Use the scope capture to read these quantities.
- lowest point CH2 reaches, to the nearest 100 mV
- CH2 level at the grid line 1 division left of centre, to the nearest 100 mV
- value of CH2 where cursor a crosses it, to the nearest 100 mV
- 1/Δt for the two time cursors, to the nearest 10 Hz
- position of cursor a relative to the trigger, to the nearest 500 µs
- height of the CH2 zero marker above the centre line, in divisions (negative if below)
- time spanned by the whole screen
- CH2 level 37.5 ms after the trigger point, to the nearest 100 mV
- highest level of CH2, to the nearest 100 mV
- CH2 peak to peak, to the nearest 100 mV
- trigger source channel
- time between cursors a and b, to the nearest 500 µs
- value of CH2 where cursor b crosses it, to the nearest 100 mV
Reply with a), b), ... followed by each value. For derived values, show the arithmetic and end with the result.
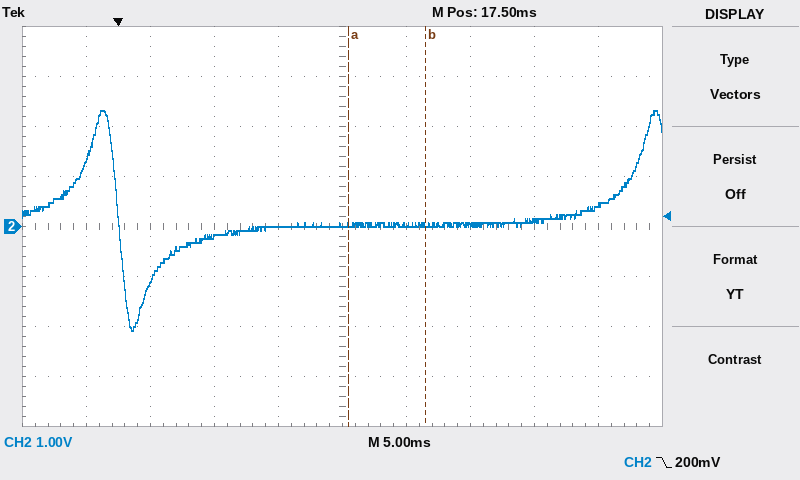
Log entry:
a) -2.1 V
b) 0.0 V
c) 0.0 V
d) 1 / 6.0 ms ≈ 170 Hz
e) +18.0 ms
f) 0.0 div
g) 50 ms
h) 400 mV
i) 2.3 V
j) 2.3 V − (-2.1 V) = 4.4 V
k) CH2
l) 6.0 ms
m) 0.0 V
